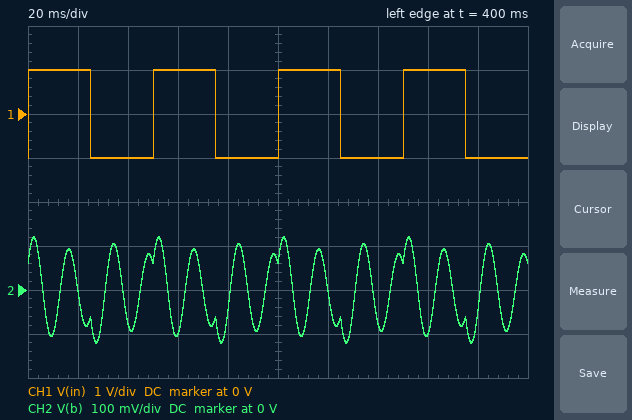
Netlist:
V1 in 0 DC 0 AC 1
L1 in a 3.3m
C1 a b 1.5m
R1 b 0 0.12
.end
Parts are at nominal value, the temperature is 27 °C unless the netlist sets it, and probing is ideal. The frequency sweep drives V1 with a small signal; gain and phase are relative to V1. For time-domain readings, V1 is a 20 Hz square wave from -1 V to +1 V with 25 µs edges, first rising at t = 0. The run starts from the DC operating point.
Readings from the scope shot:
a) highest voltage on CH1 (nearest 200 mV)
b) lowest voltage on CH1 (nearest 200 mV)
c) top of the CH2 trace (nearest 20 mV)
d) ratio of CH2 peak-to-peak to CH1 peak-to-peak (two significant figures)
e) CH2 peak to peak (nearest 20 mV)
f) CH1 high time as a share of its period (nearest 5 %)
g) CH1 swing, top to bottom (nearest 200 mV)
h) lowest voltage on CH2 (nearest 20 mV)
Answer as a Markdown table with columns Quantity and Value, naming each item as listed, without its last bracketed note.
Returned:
| Quantity | Value |
|---|---|
| highest voltage on CH1 | 1.0 V |
| lowest voltage on CH1 | -1.0 V |
| top of the CH2 trace | 120 mV |
| ratio of CH2 peak-to-peak to CH1 peak-to-peak | 0.12 |
| CH2 peak to peak | 240 mV |
| CH1 high time as a share of its period | 50 % |
| CH1 swing, top to bottom | 2.0 V |
| lowest voltage on CH2 | -120 mV |
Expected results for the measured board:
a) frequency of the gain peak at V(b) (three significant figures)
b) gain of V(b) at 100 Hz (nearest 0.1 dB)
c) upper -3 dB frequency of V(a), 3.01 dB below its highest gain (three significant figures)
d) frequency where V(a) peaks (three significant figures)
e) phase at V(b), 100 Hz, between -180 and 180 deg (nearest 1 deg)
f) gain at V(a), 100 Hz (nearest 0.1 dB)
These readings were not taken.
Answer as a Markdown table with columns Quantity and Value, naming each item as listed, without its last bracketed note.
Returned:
| Quantity | Value |
|---|---|
| frequency of the gain peak at V(b) | 71.5 Hz |
| gain of V(b) at 100 Hz | -18.6 dB |
| upper -3 dB frequency of V(a), 3.01 dB below its highest gain | 74.3 Hz |
| frequency where V(a) peaks | 71.4 Hz |
| phase at V(b), 100 Hz, between -180 and 180 deg | -83 deg |
| gain at V(a), 100 Hz | 0.4 dB |
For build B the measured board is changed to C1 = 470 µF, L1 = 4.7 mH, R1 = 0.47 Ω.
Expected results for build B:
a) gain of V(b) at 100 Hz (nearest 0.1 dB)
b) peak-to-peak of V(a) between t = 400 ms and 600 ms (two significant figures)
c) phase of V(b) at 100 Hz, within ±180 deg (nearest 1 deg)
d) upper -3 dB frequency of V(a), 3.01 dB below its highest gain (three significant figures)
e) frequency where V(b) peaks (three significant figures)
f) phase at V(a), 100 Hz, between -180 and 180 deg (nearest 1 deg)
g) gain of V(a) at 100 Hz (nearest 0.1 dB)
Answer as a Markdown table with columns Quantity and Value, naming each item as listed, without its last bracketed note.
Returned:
| Quantity | Value |
|---|---|
| gain of V(b) at 100 Hz | -2.7 dB |
| peak-to-peak of V(a) between t = 400 ms and 600 ms | 5.7 V |
| phase of V(b) at 100 Hz, within ±180 deg | 43 deg |
| upper -3 dB frequency of V(a), 3.01 dB below its highest gain | 114 Hz |
| frequency where V(b) peaks | 107 Hz |
| phase at V(a), 100 Hz, between -180 and 180 deg | -39 deg |
| gain of V(a) at 100 Hz | 14.6 dB |
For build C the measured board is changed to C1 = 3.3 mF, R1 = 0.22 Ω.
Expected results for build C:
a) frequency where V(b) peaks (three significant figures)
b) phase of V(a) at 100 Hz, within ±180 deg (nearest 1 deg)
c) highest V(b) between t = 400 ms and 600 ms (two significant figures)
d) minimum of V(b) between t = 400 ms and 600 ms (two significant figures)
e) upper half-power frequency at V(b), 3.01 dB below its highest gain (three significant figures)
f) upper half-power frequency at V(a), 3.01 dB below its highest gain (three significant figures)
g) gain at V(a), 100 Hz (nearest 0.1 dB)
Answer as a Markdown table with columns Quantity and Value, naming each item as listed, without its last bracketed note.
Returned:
| Quantity | Value |
|---|---|
| frequency where V(b) peaks | 48.2 Hz |
| phase of V(a) at 100 Hz, within ±180 deg | -148 deg |
| highest V(b) between t = 400 ms and 600 ms | 300 mV |
| minimum of V(b) between t = 400 ms and 600 ms | -300 mV |
| upper half-power frequency at V(b), 3.01 dB below its highest gain | 53.8 Hz |
| upper half-power frequency at V(a), 3.01 dB below its highest gain | 52.8 Hz |
| gain at V(a), 100 Hz | -9.6 dB |
